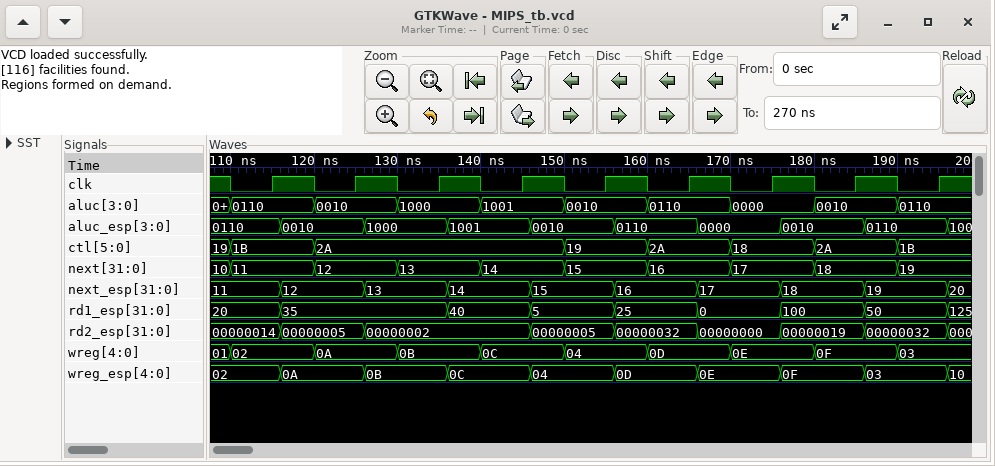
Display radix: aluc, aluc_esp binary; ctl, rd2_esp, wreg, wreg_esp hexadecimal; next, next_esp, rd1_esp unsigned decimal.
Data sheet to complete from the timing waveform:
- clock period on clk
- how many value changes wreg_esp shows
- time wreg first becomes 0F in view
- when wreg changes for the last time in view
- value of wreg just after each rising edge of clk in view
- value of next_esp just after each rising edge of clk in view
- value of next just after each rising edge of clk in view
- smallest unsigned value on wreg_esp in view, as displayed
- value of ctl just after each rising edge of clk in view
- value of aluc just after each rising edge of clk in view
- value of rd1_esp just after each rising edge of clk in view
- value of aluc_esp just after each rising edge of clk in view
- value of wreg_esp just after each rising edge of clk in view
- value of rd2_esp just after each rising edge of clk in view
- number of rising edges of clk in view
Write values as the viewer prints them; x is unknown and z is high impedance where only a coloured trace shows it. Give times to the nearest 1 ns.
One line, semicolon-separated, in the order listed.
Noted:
10 ns; 9; 180 ns; 190 ns; 02, 0A, 0B, 0C, 04, 0D, 0E, 0F, 03; 11, 12, 13, 14, 15, 16, 17, 18, 19; 11, 12, 13, 14, 15, 16, 17, 18, 19; 02; 1B, 2A, 2A, 2A, 19, 2A, 18, 2A, 1B; 0110, 0010, 1000, 1001, 0010, 0110, 0000, 0010, 0110; 20, 35, 35, 40, 5, 25, 0, 100, 50; 0110, 0010, 1000, 1001, 0010, 0110, 0000, 0010, 0110; 02, 0A, 0B, 0C, 04, 0D, 0E, 0F, 03; 00000014, 00000005, 00000002, 00000002, 00000005, 00000032, 00000000, 00000019, 00000032; 9
